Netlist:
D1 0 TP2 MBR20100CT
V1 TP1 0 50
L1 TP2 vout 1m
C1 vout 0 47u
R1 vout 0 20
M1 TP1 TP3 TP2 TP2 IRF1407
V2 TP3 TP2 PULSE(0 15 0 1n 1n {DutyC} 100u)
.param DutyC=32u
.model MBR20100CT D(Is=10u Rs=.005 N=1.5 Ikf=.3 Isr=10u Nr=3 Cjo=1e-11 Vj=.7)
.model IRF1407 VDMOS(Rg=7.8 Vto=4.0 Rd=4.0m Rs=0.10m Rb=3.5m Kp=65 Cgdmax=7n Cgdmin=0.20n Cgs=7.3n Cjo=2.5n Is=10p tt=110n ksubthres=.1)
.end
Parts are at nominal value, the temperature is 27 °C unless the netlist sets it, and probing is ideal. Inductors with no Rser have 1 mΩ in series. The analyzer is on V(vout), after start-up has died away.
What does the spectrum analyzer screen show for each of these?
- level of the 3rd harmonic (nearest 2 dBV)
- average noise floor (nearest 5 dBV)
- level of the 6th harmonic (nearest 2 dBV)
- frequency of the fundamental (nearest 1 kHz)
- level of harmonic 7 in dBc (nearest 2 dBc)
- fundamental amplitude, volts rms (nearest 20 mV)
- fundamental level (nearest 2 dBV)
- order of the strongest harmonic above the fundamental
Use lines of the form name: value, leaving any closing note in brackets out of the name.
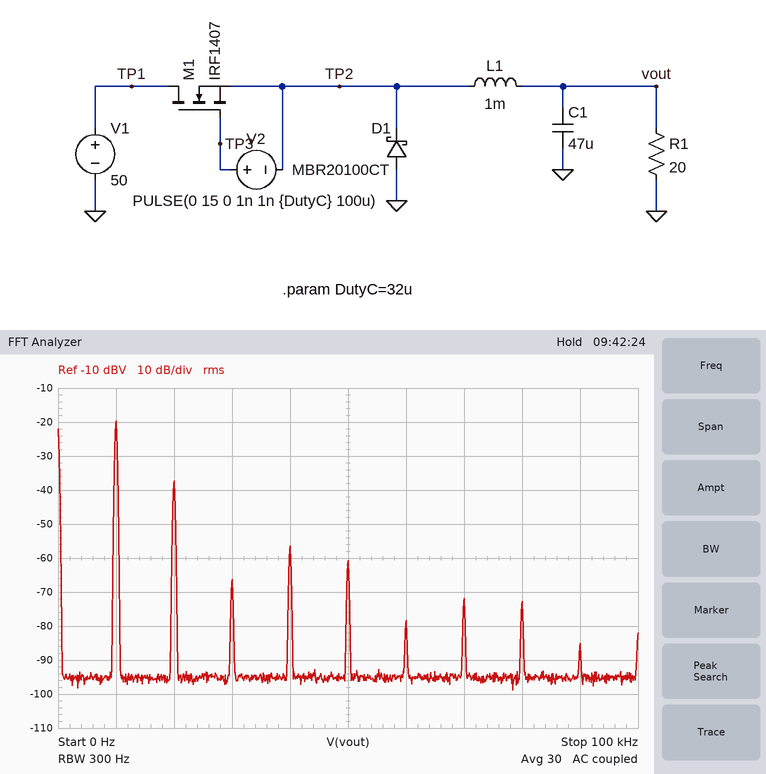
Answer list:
level of the 3rd harmonic: -66 dBV
average noise floor: -95 dBV
level of the 6th harmonic: -78 dBV
frequency of the fundamental: 10 kHz
level of harmonic 7 in dBc: -52 dBc
fundamental amplitude, volts rms: 100 mV
fundamental level: -20 dBV
order of the strongest harmonic above the fundamental: 2
